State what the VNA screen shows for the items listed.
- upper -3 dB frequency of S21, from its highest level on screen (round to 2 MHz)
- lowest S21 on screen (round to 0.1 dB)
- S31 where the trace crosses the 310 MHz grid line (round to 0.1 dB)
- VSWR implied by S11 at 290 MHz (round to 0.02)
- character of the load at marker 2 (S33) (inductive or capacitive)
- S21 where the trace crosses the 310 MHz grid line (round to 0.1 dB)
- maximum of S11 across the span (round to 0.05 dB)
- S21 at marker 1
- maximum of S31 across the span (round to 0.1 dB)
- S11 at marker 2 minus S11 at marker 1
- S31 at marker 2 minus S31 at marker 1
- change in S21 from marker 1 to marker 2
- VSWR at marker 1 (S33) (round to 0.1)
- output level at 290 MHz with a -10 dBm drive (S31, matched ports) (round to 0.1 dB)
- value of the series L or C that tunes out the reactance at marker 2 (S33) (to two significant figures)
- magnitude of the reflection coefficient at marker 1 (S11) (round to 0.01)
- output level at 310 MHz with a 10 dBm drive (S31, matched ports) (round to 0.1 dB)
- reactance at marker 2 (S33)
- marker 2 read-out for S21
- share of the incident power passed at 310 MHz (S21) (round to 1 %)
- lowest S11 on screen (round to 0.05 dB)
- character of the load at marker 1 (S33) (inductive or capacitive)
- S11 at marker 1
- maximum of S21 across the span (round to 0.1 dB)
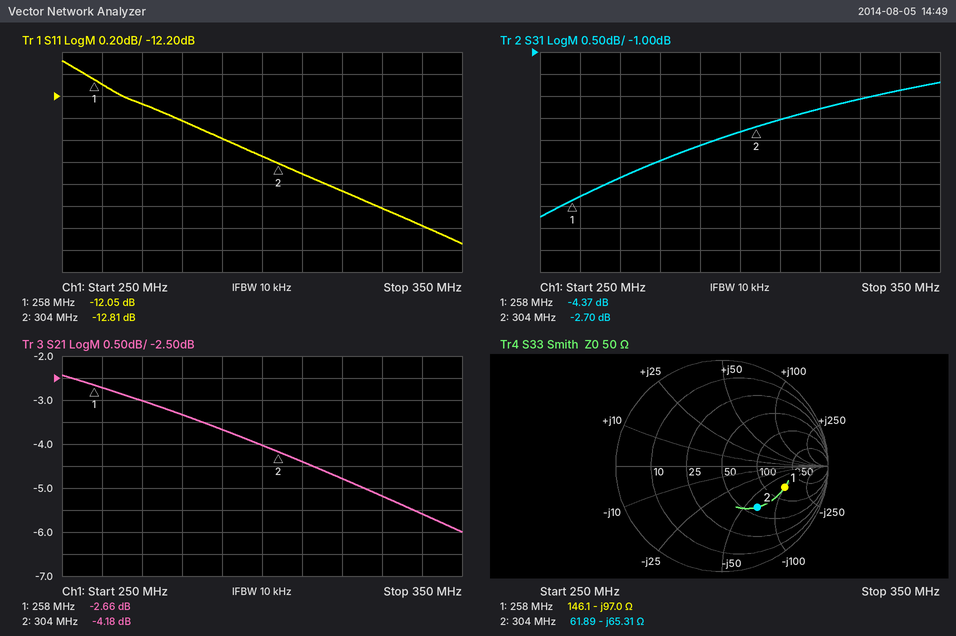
336 MHz
-6.0 dB
-2.5 dB
1.62
capacitive
-4.4 dB
-11.90 dB
-2.66 dB
-1.7 dB
-0.76 dB
1.67 dB
-1.52 dB
4.3
-13.1 dBm
34 nH
0.25
7.5 dBm
-65.31 Ω
-4.18 dB
36 %
-13.55 dB
capacitive
-12.05 dB
-2.4 dB
